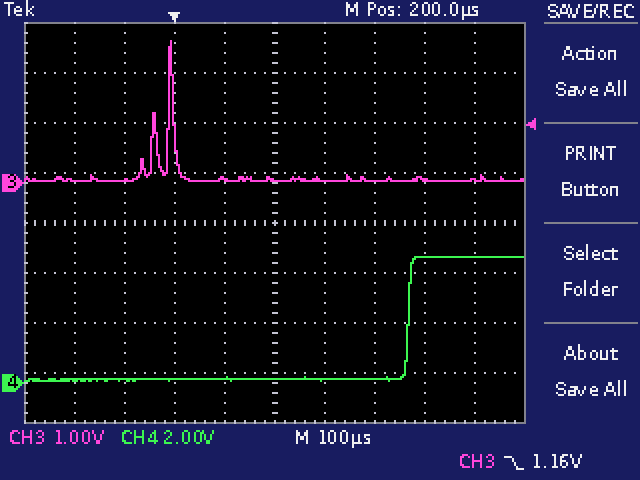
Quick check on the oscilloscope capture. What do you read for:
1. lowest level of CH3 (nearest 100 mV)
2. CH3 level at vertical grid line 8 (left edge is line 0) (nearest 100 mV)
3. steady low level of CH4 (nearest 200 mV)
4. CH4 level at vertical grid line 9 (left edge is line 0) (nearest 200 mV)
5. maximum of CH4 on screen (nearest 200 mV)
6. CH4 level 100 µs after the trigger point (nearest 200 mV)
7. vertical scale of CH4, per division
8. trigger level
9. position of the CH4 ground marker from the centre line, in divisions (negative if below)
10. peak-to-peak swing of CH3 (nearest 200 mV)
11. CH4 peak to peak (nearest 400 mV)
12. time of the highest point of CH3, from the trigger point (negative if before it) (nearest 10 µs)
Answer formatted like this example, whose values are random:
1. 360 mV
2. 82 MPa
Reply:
1. 0.0 V
2. 100 mV
3. 200 mV
4. 5.0 V
5. 5.0 V
6. 200 mV
7. 2 V
8. 1.16 V
9. -3.2 div
10. 2.8 V
11. 4.8 V
12. -10 µs
